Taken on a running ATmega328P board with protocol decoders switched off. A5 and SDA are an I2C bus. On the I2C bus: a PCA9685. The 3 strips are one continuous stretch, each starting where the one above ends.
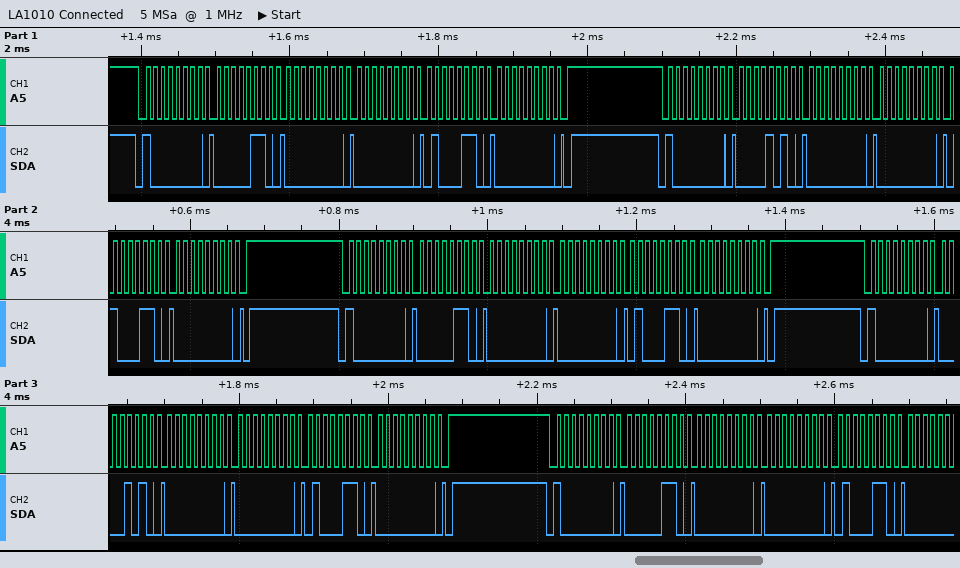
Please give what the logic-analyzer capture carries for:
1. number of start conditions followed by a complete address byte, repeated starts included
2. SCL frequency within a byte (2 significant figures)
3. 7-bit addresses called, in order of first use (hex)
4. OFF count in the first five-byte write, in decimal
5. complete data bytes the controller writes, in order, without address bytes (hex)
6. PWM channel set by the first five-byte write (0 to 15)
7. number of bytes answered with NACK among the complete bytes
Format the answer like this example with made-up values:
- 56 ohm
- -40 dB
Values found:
- 5
- 100 kHz
- 0x40
- 70
- 06 00 00 46 00 0A 00 00 46 00 06 00 00 46 00 0A 00 00 46 00 06 00 00 46
- 0
- 0
